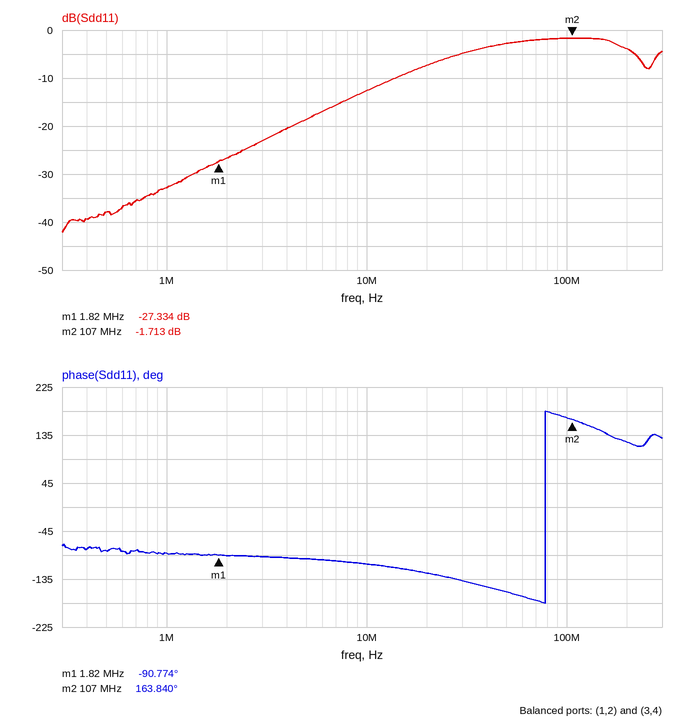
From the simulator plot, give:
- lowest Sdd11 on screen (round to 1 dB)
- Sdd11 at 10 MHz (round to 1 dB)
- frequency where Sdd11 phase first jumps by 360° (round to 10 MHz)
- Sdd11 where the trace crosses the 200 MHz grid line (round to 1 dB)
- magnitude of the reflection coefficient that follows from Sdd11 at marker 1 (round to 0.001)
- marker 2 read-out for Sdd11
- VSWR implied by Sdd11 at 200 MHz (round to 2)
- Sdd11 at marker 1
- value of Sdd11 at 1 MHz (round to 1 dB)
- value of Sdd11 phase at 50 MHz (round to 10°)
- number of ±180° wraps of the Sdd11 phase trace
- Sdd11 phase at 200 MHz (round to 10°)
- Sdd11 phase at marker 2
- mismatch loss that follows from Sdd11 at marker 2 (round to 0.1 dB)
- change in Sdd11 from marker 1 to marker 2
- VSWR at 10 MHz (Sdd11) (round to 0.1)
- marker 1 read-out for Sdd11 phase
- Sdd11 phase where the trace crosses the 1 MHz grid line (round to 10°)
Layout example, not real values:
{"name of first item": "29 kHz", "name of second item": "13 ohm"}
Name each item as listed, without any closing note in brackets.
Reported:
{"lowest Sdd11 on screen": "-42 dB", "Sdd11 at 10 MHz": "-13 dB", "frequency where Sdd11 phase first jumps by 360°": "80 MHz", "Sdd11 where the trace crosses the 200 MHz grid line": "-4 dB", "magnitude of the reflection coefficient that follows from Sdd11 at marker 1": "0.043", "marker 2 read-out for Sdd11": "-1.713 dB", "VSWR implied by Sdd11 at 200 MHz": "4", "Sdd11 at marker 1": "-27.334 dB", "value of Sdd11 at 1 MHz": "-33 dB", "value of Sdd11 phase at 50 MHz": "-160°", "number of ±180° wraps of the Sdd11 phase trace": "1", "Sdd11 phase at 200 MHz": "120°", "Sdd11 phase at marker 2": "163.840°", "mismatch loss that follows from Sdd11 at marker 2": "4.9 dB", "change in Sdd11 from marker 1 to marker 2": "25.621 dB", "VSWR at 10 MHz (Sdd11)": "1.6", "marker 1 read-out for Sdd11 phase": "-90.774°", "Sdd11 phase where the trace crosses the 1 MHz grid line": "-90°"}
